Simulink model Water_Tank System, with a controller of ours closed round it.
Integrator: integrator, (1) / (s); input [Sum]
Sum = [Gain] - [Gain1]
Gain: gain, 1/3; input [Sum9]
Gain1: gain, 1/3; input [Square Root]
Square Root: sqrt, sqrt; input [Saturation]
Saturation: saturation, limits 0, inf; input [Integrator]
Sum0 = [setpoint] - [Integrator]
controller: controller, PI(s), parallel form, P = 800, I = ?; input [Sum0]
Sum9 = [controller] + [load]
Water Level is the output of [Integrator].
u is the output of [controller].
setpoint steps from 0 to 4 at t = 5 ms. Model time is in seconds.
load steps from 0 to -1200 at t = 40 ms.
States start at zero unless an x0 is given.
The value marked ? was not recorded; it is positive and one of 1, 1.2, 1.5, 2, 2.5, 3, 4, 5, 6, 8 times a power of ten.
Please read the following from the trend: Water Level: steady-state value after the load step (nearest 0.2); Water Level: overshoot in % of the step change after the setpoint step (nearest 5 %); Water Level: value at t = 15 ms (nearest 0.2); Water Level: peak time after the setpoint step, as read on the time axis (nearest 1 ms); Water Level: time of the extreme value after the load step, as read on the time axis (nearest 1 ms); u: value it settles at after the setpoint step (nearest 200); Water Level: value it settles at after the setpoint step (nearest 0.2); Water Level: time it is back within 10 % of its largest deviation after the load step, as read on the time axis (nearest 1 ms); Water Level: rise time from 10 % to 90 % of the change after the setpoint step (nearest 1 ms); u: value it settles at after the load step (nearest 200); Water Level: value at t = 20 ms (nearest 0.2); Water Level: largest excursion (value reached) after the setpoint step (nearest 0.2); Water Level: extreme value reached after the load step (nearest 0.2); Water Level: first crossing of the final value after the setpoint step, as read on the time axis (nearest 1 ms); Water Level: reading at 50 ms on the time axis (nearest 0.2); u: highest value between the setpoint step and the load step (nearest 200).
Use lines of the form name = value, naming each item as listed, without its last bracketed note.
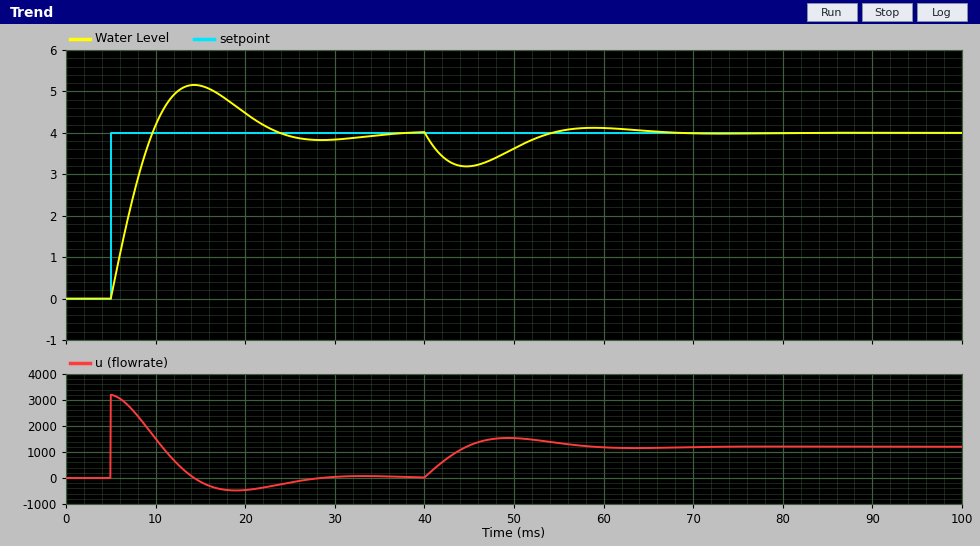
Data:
Water Level: steady-state value after the load step = 4.0
Water Level: overshoot in % of the step change after the setpoint step = 30 %
Water Level: value at t = 15 ms = 5.2
Water Level: peak time after the setpoint step, as read on the time axis = 14 ms
Water Level: time of the extreme value after the load step, as read on the time axis = 45 ms
u: value it settles at after the setpoint step = 0
Water Level: value it settles at after the setpoint step = 4.0
Water Level: time it is back within 10 % of its largest deviation after the load step, as read on the time axis = 63 ms
Water Level: rise time from 10 % to 90 % of the change after the setpoint step = 4 ms
u: value it settles at after the load step = 1200
Water Level: value at t = 20 ms = 4.4
Water Level: largest excursion (value reached) after the setpoint step = 5.2
Water Level: extreme value reached after the load step = 3.2
Water Level: first crossing of the final value after the setpoint step, as read on the time axis = 10 ms
Water Level: reading at 50 ms on the time axis = 3.6
u: highest value between the setpoint step and the load step = 3200
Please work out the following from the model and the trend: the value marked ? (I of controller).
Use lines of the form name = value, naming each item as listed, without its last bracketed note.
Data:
the value marked ? = 200000
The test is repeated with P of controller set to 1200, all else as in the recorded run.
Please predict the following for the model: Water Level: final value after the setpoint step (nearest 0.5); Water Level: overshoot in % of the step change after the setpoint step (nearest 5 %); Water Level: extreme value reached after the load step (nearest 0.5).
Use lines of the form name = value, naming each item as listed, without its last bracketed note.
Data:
Water Level: final value after the setpoint step = 4.0
Water Level: overshoot in % of the step change after the setpoint step = 20 %
Water Level: extreme value reached after the load step = 3.5
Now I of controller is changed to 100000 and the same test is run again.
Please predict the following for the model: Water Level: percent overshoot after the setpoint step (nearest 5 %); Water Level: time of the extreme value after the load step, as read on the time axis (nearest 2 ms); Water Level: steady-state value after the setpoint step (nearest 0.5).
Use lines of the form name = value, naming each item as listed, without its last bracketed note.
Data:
Water Level: percent overshoot after the setpoint step = 20 %
Water Level: time of the extreme value after the load step, as read on the time axis = 46 ms
Water Level: steady-state value after the setpoint step = 4.0
